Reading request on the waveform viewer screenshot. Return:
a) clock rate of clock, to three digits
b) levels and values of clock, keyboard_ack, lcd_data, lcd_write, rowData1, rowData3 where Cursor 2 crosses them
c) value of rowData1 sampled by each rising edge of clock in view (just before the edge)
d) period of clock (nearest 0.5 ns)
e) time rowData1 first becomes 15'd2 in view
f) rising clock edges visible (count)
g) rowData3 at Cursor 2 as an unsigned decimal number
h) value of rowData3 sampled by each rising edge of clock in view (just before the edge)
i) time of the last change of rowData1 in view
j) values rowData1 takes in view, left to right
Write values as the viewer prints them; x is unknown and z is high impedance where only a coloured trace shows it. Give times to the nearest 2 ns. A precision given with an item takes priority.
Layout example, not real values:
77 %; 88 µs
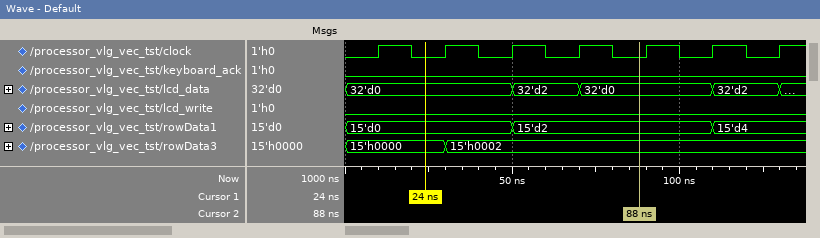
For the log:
50.0 MHz; clock=0, keyboard_ack=0, lcd_data=32'd0, lcd_write=0, rowData1=15'd2, rowData3=15'h0002; 15'd0, 15'd0, 15'd0, 15'd2, 15'd2, 15'd2, 15'd4; 20 ns; 50 ns; 7; 2; 15'h0000, 15'h0000, 15'h0002, 15'h0002, 15'h0002, 15'h0002, 15'h0002; 110 ns; 15'd0, 15'd2, 15'd4
